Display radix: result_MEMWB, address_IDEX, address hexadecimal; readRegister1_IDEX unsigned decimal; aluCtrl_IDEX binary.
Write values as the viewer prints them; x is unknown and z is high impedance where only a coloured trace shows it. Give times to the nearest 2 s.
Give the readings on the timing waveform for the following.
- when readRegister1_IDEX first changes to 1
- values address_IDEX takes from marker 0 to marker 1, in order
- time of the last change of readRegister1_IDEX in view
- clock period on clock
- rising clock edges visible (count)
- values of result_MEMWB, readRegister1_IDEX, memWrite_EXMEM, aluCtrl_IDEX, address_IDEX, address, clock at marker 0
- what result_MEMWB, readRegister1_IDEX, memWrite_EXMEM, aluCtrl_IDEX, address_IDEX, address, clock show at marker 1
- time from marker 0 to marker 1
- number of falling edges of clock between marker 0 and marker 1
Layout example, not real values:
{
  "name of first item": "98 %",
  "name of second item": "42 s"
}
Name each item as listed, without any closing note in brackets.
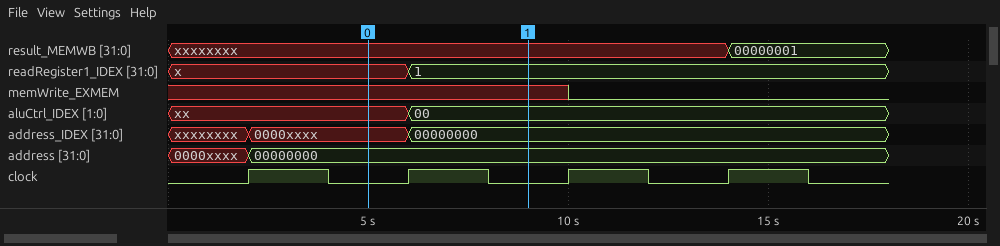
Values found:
{
  "when readRegister1_IDEX first changes to 1": "6 s",
  "values address_IDEX takes from marker 0 to marker 1, in order": "0000xxxx, 00000000",
  "time of the last change of readRegister1_IDEX in view": "6 s",
  "clock period on clock": "4 s",
  "rising clock edges visible": "4",
  "values of result_MEMWB, readRegister1_IDEX, memWrite_EXMEM, aluCtrl_IDEX, address_IDEX, address, clock at marker 0": "result_MEMWB=xxxxxxxx, readRegister1_IDEX=x, memWrite_EXMEM=x, aluCtrl_IDEX=xx, address_IDEX=0000xxxx, address=00000000, clock=0",
  "what result_MEMWB, readRegister1_IDEX, memWrite_EXMEM, aluCtrl_IDEX, address_IDEX, address, clock show at marker 1": "result_MEMWB=xxxxxxxx, readRegister1_IDEX=1, memWrite_EXMEM=x, aluCtrl_IDEX=00, address_IDEX=00000000, address=00000000, clock=0",
  "time from marker 0 to marker 1": "4 s",
  "number of falling edges of clock between marker 0 and marker 1": "1"
}
